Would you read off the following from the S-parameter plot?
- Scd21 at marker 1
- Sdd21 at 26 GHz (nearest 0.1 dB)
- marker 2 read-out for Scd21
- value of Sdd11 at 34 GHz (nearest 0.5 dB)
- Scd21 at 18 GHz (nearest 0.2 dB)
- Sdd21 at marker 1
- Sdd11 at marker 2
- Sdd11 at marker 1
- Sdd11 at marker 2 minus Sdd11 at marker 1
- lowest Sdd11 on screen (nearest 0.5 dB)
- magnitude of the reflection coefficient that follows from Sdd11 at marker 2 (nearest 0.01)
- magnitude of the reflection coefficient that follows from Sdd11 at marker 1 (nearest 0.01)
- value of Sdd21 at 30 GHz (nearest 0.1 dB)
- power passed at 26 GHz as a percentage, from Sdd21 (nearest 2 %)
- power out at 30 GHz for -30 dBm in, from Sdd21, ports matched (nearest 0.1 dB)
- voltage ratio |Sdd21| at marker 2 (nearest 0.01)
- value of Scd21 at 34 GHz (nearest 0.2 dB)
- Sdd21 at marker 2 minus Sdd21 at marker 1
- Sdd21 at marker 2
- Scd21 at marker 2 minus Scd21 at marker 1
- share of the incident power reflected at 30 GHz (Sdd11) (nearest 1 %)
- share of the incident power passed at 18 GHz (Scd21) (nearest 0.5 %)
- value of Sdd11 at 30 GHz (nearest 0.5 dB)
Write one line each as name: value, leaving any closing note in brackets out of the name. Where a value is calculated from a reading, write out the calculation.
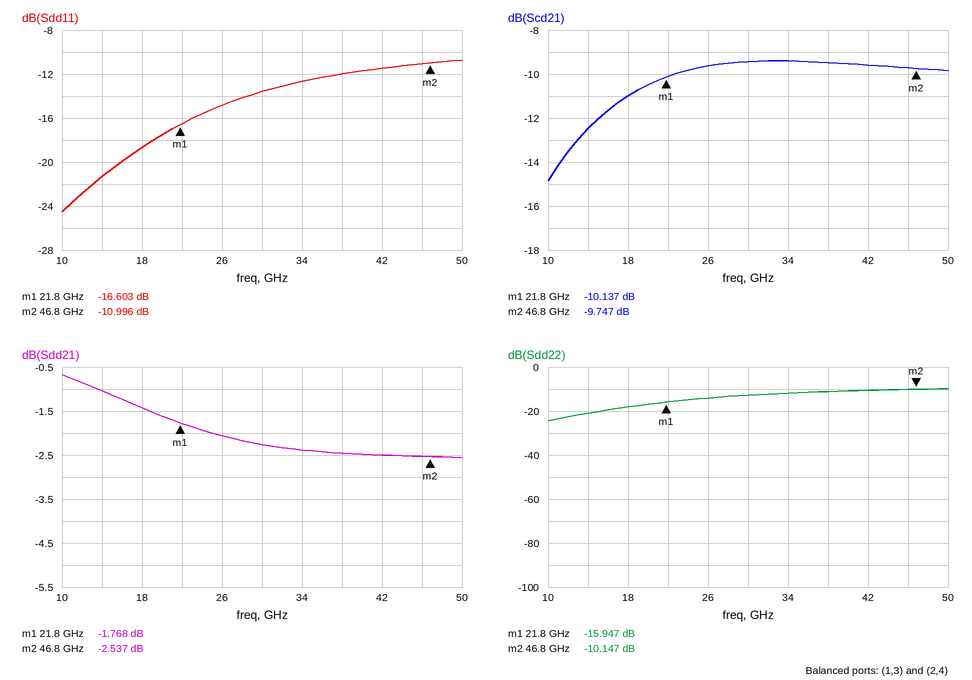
Scd21 at marker 1: -10.137 dB
Sdd21 at 26 GHz: -2.1 dB
marker 2 read-out for Scd21: -9.747 dB
value of Sdd11 at 34 GHz: -12.5 dB
Scd21 at 18 GHz: -11.0 dB
Sdd21 at marker 1: -1.768 dB
Sdd11 at marker 2: -10.996 dB
Sdd11 at marker 1: -16.603 dB
Sdd11 at marker 2 minus Sdd11 at marker 1: -10.996 − (-16.603) = 5.607 dB
lowest Sdd11 on screen: -24.5 dB
magnitude of the reflection coefficient that follows from Sdd11 at marker 2: 10^(-10.996/20) ≈ 0.28
magnitude of the reflection coefficient that follows from Sdd11 at marker 1: 10^(-16.603/20) ≈ 0.15
value of Sdd21 at 30 GHz: -2.3 dB
power passed at 26 GHz as a percentage, from Sdd21: 10^(-2.1/10) ≈ 62 %
power out at 30 GHz for -30 dBm in, from Sdd21, ports matched: -30 dBm + (-2.3 dB) = -32.3 dBm
voltage ratio |Sdd21| at marker 2: 10^(-2.537/20) ≈ 0.75
value of Scd21 at 34 GHz: -9.4 dB
Sdd21 at marker 2 minus Sdd21 at marker 1: -2.537 − (-1.768) = -0.769 dB
Sdd21 at marker 2: -2.537 dB
Scd21 at marker 2 minus Scd21 at marker 1: -9.747 − (-10.137) = 0.390 dB
share of the incident power reflected at 30 GHz (Sdd11): 10^(-13.5/10) ≈ 4 %
share of the incident power passed at 18 GHz (Scd21): 10^(-11/10) ≈ 7.94 %, so 8.0 % to the nearest 0.5 %
value of Sdd11 at 30 GHz: -13.5 dB
